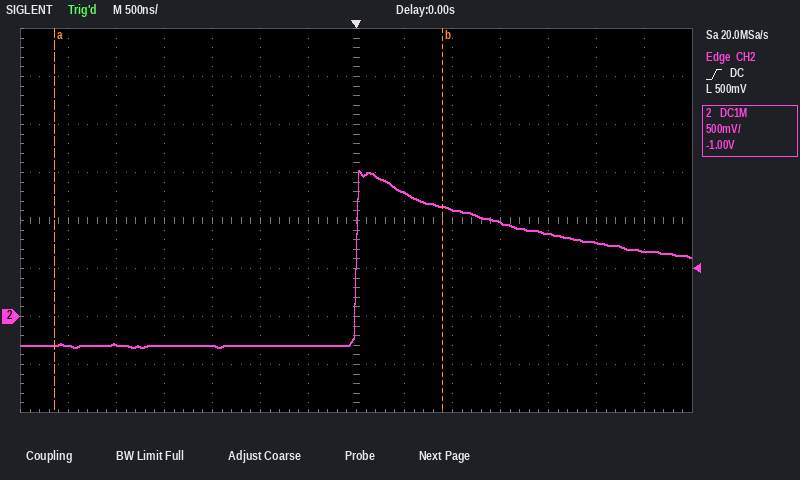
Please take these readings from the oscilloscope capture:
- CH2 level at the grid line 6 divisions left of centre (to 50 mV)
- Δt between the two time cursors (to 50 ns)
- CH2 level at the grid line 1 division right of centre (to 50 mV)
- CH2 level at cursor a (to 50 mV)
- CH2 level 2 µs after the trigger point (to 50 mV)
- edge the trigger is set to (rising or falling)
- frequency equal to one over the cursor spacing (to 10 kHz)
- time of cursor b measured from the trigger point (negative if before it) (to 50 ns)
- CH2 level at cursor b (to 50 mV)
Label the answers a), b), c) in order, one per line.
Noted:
a) -300 mV
b) 4.05 µs
c) 1.30 V
d) -300 mV
e) 850 mV
f) rising
g) 250 kHz
h) +900 ns
i) 1.15 V
